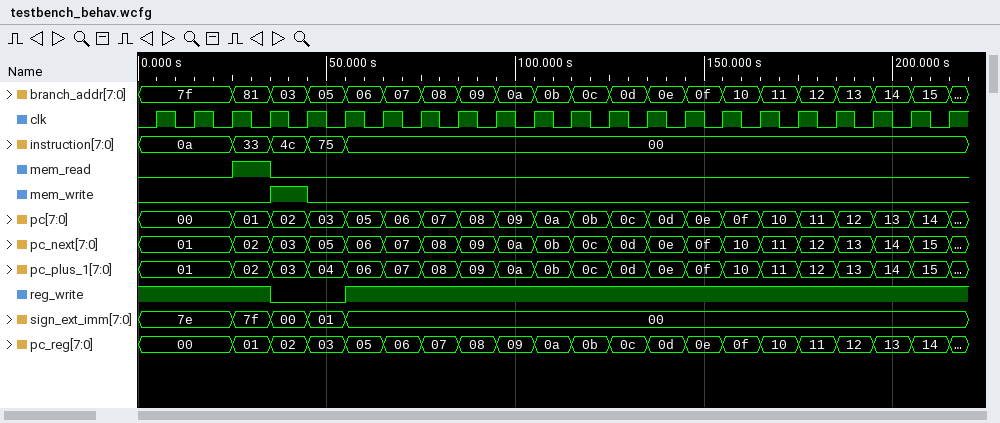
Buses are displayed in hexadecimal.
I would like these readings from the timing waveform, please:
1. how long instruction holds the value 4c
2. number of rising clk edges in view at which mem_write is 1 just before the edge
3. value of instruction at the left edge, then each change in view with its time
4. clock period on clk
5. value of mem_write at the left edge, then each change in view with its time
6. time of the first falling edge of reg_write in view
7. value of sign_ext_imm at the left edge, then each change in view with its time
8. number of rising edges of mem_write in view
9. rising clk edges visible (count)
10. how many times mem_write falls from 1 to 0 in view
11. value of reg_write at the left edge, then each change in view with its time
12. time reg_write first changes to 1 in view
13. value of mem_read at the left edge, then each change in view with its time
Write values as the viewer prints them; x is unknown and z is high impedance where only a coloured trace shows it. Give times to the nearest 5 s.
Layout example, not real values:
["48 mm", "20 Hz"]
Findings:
["10 s", "1", "0a, 33 at 25 s, 4c at 35 s, 75 at 45 s, 00 at 55 s", "10 s", "0, 1 at 35 s, 0 at 45 s", "35 s", "7e, 7f at 25 s, 00 at 35 s, 01 at 45 s, 00 at 55 s", "1", "22", "1", "1, 0 at 35 s, 1 at 55 s", "55 s", "0, 1 at 25 s, 0 at 35 s"]
